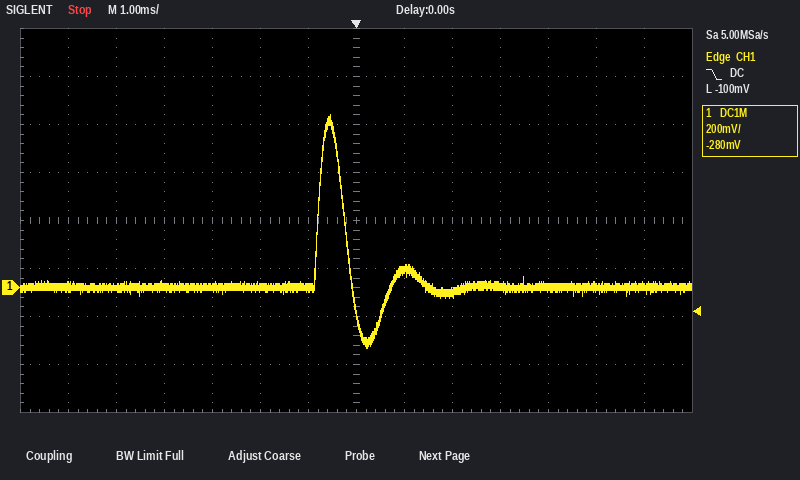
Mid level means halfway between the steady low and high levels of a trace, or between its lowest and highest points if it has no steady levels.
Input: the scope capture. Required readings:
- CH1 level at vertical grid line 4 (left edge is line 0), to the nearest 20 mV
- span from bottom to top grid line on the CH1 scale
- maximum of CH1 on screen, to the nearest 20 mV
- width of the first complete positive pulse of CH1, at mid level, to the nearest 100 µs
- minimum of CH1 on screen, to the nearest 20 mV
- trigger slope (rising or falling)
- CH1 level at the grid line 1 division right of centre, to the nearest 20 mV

0 mV
1.6 V
720 mV
600 µs
-240 mV
falling
80 mV
